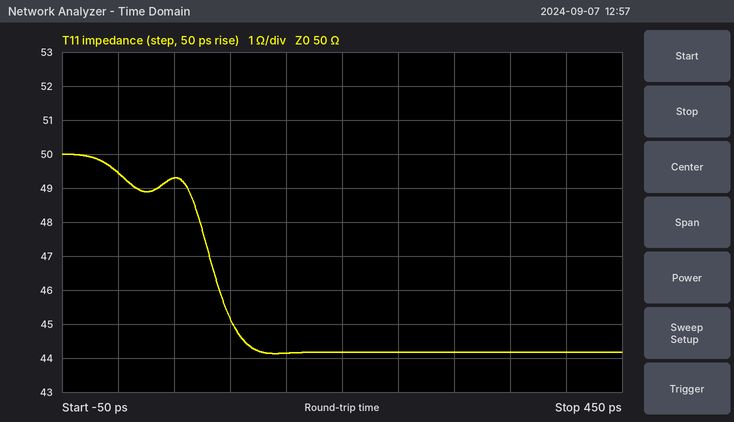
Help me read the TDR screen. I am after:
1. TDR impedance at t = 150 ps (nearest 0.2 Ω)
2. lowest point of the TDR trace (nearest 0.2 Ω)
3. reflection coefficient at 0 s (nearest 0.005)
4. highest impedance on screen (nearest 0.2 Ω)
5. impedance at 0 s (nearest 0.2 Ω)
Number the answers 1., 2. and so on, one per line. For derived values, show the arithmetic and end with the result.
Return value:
1. 44.2 Ω
2. 44.2 Ω
3. (49.4 − 50)/(49.4 + 50) ≈ -0.00604, so -0.005 to the nearest 0.005
4. 50.0 Ω
5. 49.4 Ω
